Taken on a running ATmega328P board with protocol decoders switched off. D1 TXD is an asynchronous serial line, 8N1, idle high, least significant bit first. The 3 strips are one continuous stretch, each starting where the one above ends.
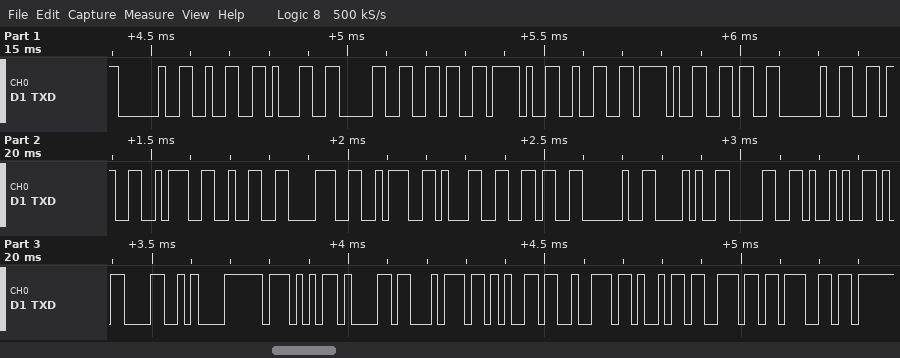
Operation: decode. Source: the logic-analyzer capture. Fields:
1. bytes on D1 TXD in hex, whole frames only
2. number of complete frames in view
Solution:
20 32 31 30 36 2F 32 2F 36 20 36 3A 32 38 3A 31 36 20 28 30 29 0D 0A 57 61 74 65 72 69 6E 67
31
